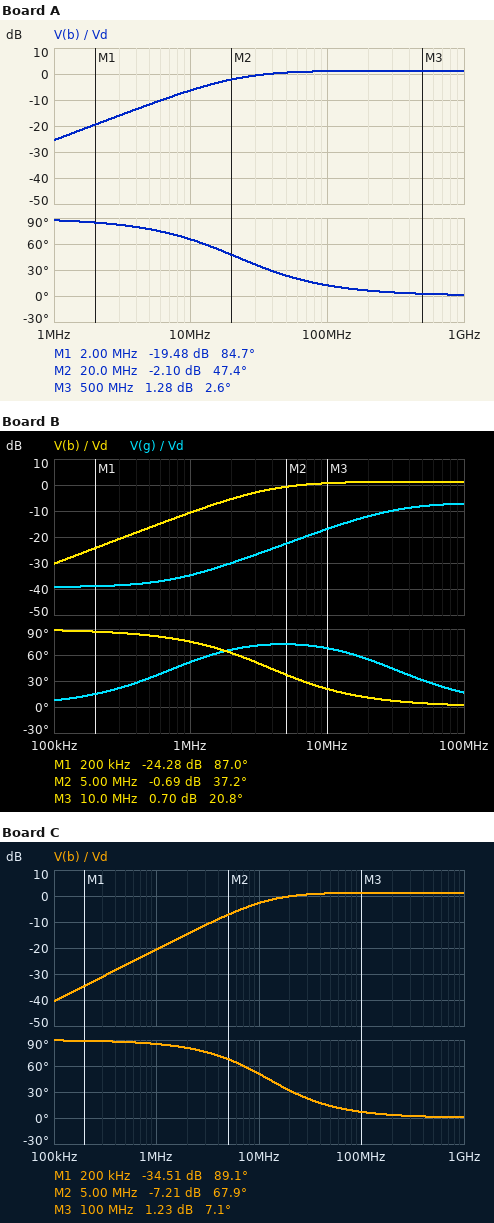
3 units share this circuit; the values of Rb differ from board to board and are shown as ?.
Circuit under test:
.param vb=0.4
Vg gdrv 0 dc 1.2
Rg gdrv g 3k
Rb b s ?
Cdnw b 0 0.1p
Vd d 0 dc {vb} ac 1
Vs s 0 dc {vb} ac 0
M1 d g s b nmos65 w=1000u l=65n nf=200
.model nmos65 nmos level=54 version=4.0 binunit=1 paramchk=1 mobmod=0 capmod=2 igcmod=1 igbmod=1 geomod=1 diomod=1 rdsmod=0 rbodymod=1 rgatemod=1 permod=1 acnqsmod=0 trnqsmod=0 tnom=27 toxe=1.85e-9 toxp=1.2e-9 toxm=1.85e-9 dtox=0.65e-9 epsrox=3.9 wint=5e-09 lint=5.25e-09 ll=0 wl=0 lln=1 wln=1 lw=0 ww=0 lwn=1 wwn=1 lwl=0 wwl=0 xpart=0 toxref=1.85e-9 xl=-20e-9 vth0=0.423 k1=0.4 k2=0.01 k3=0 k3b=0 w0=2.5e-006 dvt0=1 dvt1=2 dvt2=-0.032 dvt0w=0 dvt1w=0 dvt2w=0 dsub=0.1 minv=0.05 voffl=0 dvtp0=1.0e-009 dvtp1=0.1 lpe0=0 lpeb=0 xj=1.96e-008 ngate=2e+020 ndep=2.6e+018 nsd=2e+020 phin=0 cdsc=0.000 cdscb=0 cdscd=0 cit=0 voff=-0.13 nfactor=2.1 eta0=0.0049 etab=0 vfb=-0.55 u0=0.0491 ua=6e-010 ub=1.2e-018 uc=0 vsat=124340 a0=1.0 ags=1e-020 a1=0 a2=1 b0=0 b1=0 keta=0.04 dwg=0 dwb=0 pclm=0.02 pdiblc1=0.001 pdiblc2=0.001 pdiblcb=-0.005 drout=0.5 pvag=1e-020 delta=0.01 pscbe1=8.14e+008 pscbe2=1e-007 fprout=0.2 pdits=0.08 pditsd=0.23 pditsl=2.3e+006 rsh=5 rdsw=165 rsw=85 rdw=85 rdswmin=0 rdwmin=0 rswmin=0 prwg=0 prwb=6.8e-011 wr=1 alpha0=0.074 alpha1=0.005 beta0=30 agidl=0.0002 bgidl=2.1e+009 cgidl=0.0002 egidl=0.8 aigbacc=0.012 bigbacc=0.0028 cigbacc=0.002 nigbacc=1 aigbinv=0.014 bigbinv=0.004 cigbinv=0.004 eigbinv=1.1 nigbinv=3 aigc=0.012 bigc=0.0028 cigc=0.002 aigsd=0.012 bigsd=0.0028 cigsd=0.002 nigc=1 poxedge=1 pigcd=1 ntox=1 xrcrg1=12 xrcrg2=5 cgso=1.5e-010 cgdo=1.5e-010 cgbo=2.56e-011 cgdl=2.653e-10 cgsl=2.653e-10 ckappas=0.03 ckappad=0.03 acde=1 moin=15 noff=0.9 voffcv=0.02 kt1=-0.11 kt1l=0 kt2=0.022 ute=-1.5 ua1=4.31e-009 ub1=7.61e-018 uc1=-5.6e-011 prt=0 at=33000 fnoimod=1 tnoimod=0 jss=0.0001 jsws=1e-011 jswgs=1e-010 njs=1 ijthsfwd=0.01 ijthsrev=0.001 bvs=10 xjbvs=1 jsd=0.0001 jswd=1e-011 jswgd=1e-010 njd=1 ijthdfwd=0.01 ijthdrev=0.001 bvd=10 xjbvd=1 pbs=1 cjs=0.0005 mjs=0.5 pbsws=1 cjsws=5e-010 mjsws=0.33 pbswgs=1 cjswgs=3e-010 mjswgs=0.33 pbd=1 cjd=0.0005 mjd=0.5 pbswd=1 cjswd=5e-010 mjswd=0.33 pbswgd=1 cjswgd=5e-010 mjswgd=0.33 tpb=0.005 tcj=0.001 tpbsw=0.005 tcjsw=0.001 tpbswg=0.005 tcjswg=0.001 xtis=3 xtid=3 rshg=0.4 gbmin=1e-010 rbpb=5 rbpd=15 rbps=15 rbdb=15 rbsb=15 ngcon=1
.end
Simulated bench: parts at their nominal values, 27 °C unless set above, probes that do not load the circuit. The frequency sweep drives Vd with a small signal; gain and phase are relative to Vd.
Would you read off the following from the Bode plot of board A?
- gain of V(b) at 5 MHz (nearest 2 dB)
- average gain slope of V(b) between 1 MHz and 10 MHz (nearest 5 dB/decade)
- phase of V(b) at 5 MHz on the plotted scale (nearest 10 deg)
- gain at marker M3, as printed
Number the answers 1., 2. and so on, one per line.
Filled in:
1. -12 dB
2. 20 dB/decade
3. 80 deg
4. 1.28 dB
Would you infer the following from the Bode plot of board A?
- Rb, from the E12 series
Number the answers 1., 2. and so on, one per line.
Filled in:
1. 6.8 kΩ
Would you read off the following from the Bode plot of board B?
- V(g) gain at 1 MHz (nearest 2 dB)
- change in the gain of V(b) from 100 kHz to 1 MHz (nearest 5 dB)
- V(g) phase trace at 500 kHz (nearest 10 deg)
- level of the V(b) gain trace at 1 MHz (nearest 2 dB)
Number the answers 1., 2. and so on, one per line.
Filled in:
1. -34 dB
2. 20 dB
3. 30 deg
4. -10 dB
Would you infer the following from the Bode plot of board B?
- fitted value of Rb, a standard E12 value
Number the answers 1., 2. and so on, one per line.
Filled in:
1. 39 kΩ
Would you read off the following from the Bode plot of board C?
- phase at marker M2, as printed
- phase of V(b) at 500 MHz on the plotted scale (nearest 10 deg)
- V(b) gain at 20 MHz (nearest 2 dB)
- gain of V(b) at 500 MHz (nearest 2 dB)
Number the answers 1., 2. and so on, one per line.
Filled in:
1. 67.9 deg
2. 0 deg
3. 0 dB
4. 2 dB
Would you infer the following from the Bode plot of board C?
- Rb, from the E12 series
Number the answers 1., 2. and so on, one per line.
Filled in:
1. 12 kΩ
